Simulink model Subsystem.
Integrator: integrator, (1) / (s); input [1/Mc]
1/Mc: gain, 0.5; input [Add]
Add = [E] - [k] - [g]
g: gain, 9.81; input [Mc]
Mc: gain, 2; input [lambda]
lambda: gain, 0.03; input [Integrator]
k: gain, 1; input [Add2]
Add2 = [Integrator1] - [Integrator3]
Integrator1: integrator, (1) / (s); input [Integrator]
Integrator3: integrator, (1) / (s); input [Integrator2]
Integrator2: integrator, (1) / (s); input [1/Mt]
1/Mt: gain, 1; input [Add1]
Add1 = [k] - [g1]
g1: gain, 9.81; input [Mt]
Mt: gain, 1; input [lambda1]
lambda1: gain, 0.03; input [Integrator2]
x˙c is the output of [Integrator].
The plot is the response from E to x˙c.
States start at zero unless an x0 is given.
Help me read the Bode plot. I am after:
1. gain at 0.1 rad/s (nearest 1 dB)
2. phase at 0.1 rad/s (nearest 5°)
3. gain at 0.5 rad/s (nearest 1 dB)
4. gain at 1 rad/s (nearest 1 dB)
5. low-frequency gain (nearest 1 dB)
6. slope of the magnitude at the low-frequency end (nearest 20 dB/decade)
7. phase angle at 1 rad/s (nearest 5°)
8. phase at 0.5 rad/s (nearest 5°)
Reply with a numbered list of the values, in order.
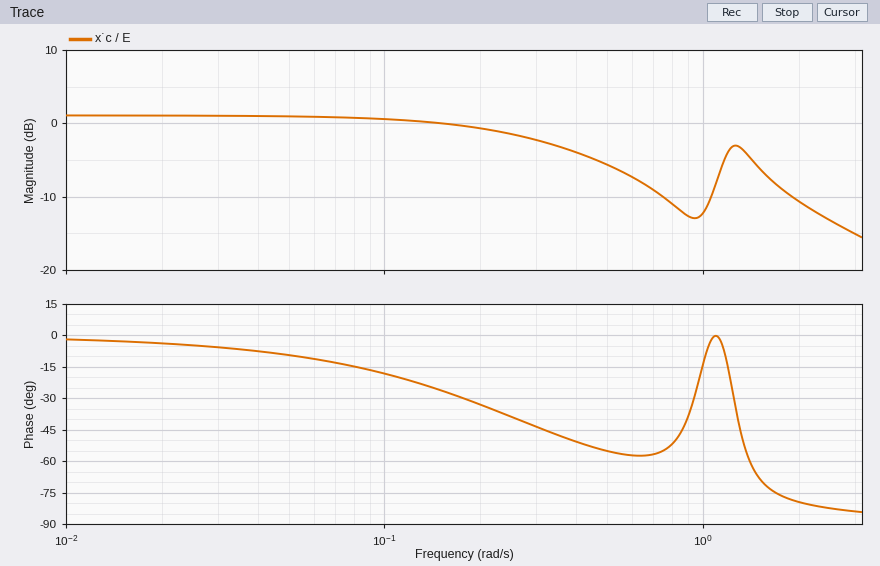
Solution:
1. 1 dB
2. -20°
3. -6 dB
4. -12 dB
5. 1 dB
6. 0 dB/decade
7. -15°
8. -55°
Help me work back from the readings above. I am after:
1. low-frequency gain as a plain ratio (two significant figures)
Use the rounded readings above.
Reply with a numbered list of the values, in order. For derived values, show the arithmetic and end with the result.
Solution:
1. 10^(1 / 20) = 1.1
